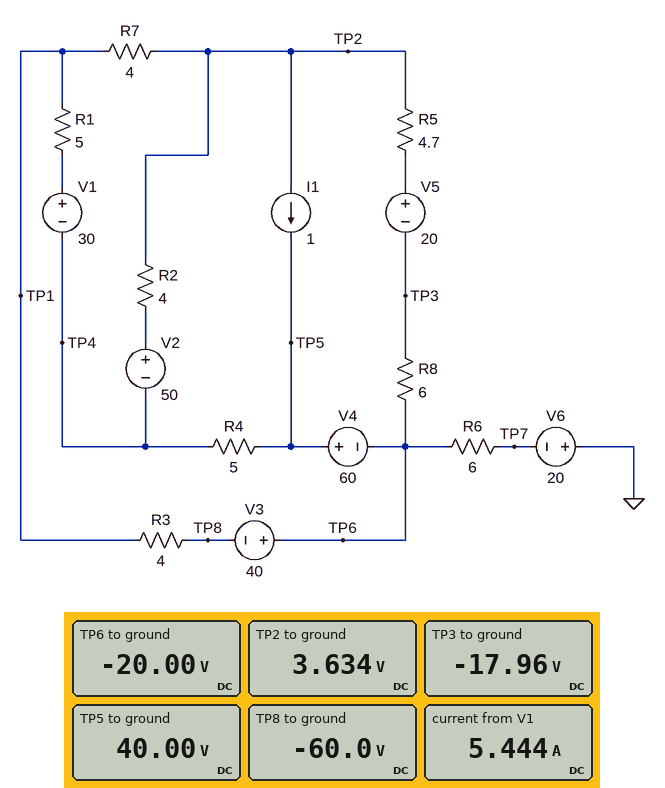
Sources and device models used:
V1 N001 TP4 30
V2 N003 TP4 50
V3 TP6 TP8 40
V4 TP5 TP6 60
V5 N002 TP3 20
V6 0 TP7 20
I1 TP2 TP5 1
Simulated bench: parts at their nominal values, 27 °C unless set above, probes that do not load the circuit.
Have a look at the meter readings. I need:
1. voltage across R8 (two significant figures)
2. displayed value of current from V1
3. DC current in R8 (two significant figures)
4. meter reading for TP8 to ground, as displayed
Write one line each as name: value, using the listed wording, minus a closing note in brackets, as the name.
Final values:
voltage across R8: 2.0 V
displayed value of current from V1: 5.444 A
DC current in R8: 340 mA
meter reading for TP8 to ground, as displayed: -60.0 V
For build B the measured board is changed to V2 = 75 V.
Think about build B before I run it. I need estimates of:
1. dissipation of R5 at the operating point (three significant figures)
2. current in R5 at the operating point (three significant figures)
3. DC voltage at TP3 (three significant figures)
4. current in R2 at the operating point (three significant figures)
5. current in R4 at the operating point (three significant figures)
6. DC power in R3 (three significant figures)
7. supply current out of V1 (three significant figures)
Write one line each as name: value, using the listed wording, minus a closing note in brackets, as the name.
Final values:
dissipation of R5 at the operating point: 6.22 W
current in R5 at the operating point: 1.15 A
DC voltage at TP3: -13.1 V
current in R2 at the operating point: 9.19 A
current in R4 at the operating point: 13.2 A
DC power in R3: 487 W
supply current out of V1: 3.99 A
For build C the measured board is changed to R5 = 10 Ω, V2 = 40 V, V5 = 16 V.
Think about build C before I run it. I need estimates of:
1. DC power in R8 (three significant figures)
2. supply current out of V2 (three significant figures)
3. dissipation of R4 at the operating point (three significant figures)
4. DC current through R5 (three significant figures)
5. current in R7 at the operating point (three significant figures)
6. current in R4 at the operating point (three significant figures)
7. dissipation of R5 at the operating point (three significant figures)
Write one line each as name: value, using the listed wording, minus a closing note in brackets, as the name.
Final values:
DC power in R8: 262 mW
supply current out of V2: 5.62 A
dissipation of R4 at the operating point: 677 W
DC current through R5: 209 mA
current in R7 at the operating point: 4.41 A
current in R4 at the operating point: 11.6 A
dissipation of R5 at the operating point: 437 mW
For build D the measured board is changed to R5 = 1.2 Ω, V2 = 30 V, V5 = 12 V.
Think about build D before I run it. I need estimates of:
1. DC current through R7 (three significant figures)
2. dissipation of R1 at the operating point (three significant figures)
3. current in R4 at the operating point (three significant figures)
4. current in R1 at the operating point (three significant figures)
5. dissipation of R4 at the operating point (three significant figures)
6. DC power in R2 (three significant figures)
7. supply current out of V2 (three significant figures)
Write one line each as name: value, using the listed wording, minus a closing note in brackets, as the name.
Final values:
DC current through R7: 3.47 A
dissipation of R1 at the operating point: 217 W
current in R4 at the operating point: 11.4 A
current in R1 at the operating point: 6.59 A
dissipation of R4 at the operating point: 645 W
DC power in R2: 90.9 W
supply current out of V2: 4.77 A
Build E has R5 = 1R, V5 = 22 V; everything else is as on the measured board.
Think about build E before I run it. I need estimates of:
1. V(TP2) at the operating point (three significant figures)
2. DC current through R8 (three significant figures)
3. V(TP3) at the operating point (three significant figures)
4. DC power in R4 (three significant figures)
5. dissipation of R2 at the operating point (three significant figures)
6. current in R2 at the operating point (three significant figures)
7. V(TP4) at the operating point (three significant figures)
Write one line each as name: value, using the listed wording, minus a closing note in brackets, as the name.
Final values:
V(TP2) at the operating point: 3.91 V
DC current through R8: 273 mA
V(TP3) at the operating point: -18.4 V
DC power in R4: 718 W
dissipation of R2 at the operating point: 171 W
current in R2 at the operating point: 6.54 A
V(TP4) at the operating point: -19.9 V
